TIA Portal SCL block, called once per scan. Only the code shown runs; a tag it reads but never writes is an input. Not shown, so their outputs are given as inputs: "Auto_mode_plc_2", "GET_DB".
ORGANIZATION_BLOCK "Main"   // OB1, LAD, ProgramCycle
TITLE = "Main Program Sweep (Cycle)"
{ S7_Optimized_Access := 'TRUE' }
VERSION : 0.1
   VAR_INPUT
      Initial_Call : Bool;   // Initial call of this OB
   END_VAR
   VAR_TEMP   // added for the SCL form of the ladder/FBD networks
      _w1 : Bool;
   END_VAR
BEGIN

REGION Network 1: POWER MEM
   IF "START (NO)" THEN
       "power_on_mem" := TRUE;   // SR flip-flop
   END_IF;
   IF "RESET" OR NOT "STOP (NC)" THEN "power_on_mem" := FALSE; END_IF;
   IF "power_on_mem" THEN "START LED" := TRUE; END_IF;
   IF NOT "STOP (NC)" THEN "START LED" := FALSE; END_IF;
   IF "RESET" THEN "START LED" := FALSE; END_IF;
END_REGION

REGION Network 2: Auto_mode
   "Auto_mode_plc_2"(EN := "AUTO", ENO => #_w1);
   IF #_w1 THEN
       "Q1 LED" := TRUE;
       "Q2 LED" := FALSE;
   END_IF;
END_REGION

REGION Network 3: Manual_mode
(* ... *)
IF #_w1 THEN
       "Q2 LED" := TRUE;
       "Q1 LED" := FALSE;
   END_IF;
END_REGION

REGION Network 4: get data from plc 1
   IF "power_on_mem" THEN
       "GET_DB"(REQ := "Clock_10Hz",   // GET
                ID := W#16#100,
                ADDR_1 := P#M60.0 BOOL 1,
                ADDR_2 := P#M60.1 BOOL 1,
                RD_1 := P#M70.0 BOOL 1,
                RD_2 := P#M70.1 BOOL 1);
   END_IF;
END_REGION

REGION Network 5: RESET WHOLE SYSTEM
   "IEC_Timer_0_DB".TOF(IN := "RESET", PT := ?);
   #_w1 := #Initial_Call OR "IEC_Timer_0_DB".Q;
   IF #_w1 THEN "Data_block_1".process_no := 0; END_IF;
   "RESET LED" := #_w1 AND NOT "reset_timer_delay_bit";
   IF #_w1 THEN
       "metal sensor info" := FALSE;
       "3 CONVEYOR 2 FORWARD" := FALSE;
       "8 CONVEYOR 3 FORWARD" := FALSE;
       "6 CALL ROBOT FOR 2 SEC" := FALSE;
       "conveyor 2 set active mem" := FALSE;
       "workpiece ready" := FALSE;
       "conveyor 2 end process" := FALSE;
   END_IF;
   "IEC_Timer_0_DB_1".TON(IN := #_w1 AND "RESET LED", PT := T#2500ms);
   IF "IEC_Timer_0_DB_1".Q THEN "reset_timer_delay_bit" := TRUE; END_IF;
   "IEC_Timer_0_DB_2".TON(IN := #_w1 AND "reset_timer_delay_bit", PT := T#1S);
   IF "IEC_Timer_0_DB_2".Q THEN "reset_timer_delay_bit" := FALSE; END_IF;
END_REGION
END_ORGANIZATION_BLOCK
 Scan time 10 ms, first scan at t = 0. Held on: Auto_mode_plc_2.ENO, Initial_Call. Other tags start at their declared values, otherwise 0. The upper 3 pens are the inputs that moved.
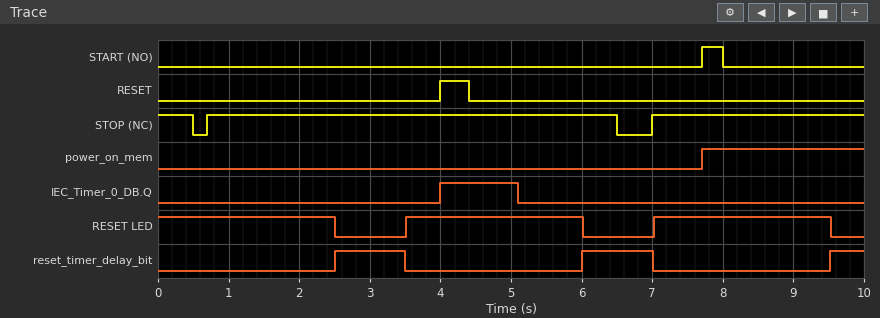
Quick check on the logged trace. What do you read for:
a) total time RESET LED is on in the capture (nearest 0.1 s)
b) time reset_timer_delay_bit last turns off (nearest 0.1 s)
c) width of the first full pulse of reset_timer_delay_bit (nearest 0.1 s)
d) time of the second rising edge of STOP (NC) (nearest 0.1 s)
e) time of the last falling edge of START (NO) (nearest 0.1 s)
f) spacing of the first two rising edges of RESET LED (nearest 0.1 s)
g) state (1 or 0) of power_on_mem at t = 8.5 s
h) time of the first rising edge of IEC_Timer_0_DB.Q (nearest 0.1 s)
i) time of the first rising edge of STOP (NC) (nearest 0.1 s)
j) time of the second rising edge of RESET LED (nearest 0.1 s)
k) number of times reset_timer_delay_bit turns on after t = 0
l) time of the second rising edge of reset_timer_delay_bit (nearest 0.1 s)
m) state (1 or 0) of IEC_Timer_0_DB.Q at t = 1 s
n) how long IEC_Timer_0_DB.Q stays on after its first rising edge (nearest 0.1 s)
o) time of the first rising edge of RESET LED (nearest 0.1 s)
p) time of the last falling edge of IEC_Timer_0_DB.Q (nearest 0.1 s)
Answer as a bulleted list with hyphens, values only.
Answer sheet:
- 7.5 s
- 7.0 s
- 1.0 s
- 7.0 s
- 8.0 s
- 3.5 s
- 1
- 4.0 s
- 0.7 s
- 7.0 s
- 3
- 6.0 s
- 0
- 1.1 s
- 3.5 s
- 5.1 s
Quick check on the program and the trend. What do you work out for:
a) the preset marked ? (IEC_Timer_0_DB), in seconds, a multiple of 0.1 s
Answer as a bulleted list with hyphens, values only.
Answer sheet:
- 0.7 s
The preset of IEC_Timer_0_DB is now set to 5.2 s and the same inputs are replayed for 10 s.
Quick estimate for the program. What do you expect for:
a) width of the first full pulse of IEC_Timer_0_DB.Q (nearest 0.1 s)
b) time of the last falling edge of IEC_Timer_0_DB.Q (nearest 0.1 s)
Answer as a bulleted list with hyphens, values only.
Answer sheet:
- 5.6 s
- 9.6 s
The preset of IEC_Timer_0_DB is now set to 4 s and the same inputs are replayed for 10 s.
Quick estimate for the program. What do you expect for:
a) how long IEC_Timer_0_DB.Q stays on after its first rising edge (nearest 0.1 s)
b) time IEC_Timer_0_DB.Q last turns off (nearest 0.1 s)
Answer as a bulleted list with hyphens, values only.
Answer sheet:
- 4.4 s
- 8.4 s
